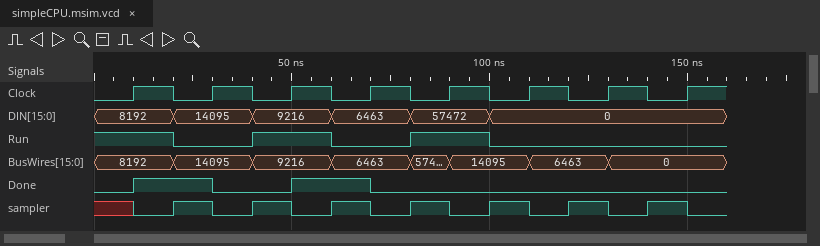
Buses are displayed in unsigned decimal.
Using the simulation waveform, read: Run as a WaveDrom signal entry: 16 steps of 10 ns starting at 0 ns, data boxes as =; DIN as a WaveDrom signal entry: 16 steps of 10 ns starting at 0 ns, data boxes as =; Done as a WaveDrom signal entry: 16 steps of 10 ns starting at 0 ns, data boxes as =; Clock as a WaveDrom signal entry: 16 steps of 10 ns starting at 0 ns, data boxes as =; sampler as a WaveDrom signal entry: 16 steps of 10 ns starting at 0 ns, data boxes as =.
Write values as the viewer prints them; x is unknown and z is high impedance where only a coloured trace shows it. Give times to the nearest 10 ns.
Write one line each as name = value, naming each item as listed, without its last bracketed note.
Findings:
Run as a WaveDrom signal entry: 16 steps of 10 ns starting at 0 ns, data boxes as = = {name: 'Run', wave: '1.0.1.0.1.0.....'}
DIN as a WaveDrom signal entry: 16 steps of 10 ns starting at 0 ns, data boxes as = = {name: 'DIN', wave: '=.=.=.=.=.=.....', data: '8192 14095 9216 6463 57472 0'}
Done as a WaveDrom signal entry: 16 steps of 10 ns starting at 0 ns, data boxes as = = {name: 'Done', wave: '01.0.1.0........'}
Clock as a WaveDrom signal entry: 16 steps of 10 ns starting at 0 ns, data boxes as = = {name: 'Clock', wave: '0101010101010101'}
sampler as a WaveDrom signal entry: 16 steps of 10 ns starting at 0 ns, data boxes as = = {name: 'sampler', wave: 'x010101010101010'}
